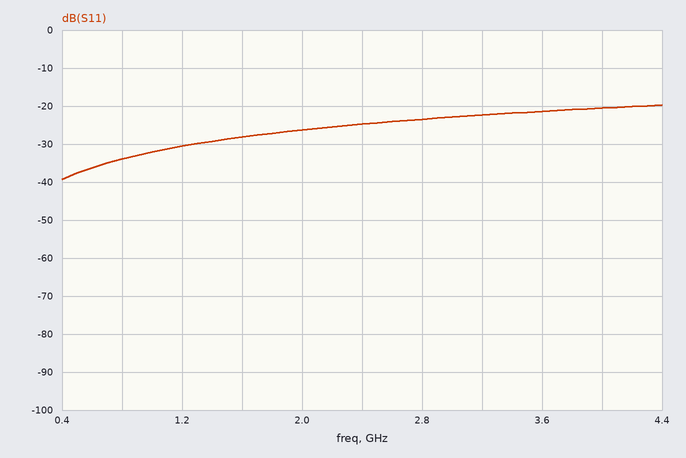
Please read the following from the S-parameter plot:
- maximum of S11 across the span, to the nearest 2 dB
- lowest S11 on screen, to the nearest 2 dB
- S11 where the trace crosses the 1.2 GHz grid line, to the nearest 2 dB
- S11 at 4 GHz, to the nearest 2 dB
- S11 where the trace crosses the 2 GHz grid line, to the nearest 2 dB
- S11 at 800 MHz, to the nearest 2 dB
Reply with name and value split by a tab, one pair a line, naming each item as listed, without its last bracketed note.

maximum of S11 across the span, to the nearest 2 dB	-20 dB
lowest S11 on screen, to the nearest 2 dB	-40 dB
S11 where the trace crosses the 1.2 GHz grid line, to the nearest 2 dB	-30 dB
S11 at 4 GHz, to the nearest 2 dB	-20 dB
S11 where the trace crosses the 2 GHz grid line, to the nearest 2 dB	-26 dB
S11 at 800 MHz, to the nearest 2 dB	-34 dB
